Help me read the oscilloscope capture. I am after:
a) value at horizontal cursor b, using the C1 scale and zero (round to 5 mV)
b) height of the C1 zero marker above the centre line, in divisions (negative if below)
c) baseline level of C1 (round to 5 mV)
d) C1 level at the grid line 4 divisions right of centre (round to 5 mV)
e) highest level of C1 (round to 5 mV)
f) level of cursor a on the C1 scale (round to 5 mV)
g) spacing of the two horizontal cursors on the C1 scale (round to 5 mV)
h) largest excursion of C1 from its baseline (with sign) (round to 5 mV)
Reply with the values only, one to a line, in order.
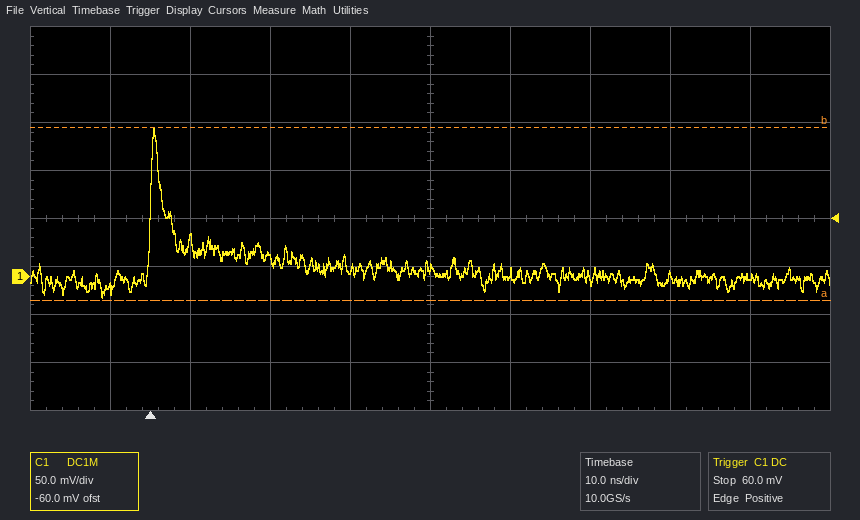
155 mV
-1.2 div
0 mV
0 mV
155 mV
-25 mV
180 mV
+155 mV
